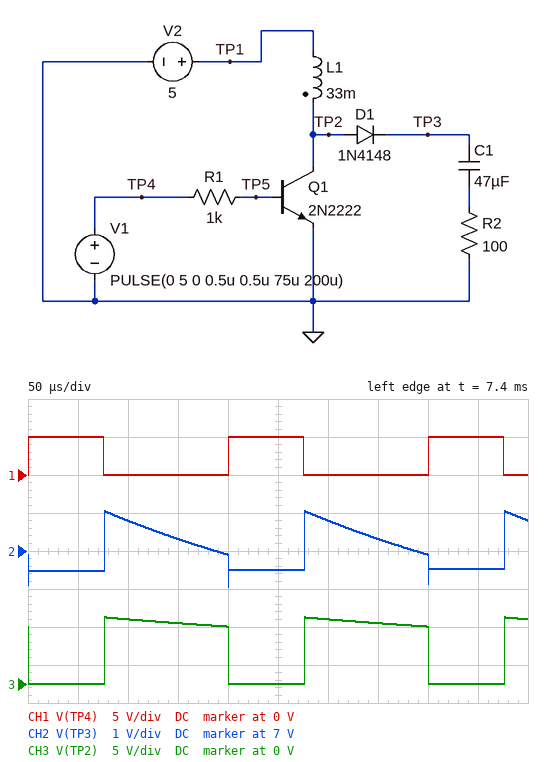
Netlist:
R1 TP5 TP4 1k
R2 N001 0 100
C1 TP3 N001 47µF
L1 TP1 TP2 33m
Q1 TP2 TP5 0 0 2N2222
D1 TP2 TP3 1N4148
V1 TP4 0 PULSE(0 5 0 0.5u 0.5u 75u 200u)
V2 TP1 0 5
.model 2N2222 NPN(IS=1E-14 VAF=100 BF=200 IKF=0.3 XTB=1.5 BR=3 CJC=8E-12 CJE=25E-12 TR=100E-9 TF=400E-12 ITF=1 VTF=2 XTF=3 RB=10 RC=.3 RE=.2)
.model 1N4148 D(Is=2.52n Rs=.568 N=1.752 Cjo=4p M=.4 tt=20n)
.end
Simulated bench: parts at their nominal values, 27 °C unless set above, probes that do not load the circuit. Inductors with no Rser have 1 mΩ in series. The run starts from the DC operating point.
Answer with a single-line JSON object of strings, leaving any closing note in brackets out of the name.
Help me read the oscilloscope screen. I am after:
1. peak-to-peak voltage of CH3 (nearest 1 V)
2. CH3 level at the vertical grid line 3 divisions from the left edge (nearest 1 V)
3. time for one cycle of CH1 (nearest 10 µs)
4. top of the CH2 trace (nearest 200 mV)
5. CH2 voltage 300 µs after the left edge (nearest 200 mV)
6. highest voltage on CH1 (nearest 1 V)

{"peak-to-peak voltage of CH3": "9 V", "CH3 level at the vertical grid line 3 divisions from the left edge": "8 V", "time for one cycle of CH1": "200 µs", "top of the CH2 trace": "8.0 V", "CH2 voltage 300 µs after the left edge": "7.8 V", "highest voltage on CH1": "5 V"}
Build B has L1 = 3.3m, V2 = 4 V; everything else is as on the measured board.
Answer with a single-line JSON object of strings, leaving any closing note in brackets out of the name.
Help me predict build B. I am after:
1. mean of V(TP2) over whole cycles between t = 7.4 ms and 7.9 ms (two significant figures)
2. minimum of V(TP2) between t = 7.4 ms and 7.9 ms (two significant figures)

{"mean of V(TP2) over whole cycles between t = 7.4 ms and 7.9 ms": "4.0 V", "minimum of V(TP2) between t = 7.4 ms and 7.9 ms": "12 mV"}
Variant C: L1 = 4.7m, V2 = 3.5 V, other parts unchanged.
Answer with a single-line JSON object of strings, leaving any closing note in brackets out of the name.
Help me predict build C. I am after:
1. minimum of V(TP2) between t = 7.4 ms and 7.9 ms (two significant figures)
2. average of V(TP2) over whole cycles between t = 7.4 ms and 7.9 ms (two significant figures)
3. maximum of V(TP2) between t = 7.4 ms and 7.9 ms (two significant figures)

{"minimum of V(TP2) between t = 7.4 ms and 7.9 ms": "11 mV", "average of V(TP2) over whole cycles between t = 7.4 ms and 7.9 ms": "3.5 V", "maximum of V(TP2) between t = 7.4 ms and 7.9 ms": "11 V"}
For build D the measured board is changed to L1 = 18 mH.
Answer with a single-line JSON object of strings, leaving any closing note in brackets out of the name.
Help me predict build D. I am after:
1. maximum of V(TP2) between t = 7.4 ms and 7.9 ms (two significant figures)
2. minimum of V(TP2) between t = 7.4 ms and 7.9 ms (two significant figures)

{"maximum of V(TP2) between t = 7.4 ms and 7.9 ms": "9.4 V", "minimum of V(TP2) between t = 7.4 ms and 7.9 ms": "9.5 mV"}
